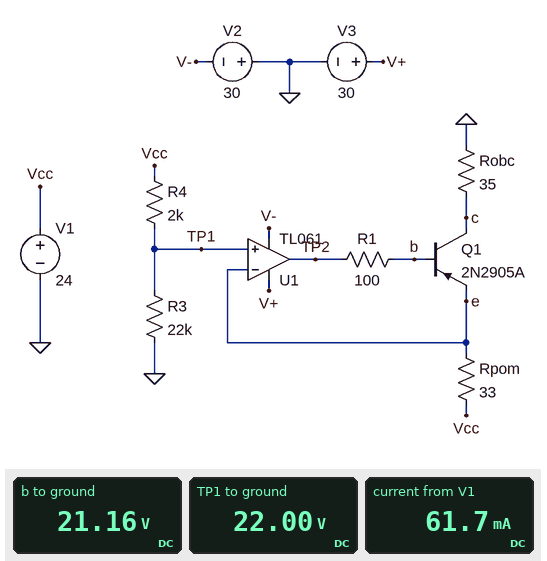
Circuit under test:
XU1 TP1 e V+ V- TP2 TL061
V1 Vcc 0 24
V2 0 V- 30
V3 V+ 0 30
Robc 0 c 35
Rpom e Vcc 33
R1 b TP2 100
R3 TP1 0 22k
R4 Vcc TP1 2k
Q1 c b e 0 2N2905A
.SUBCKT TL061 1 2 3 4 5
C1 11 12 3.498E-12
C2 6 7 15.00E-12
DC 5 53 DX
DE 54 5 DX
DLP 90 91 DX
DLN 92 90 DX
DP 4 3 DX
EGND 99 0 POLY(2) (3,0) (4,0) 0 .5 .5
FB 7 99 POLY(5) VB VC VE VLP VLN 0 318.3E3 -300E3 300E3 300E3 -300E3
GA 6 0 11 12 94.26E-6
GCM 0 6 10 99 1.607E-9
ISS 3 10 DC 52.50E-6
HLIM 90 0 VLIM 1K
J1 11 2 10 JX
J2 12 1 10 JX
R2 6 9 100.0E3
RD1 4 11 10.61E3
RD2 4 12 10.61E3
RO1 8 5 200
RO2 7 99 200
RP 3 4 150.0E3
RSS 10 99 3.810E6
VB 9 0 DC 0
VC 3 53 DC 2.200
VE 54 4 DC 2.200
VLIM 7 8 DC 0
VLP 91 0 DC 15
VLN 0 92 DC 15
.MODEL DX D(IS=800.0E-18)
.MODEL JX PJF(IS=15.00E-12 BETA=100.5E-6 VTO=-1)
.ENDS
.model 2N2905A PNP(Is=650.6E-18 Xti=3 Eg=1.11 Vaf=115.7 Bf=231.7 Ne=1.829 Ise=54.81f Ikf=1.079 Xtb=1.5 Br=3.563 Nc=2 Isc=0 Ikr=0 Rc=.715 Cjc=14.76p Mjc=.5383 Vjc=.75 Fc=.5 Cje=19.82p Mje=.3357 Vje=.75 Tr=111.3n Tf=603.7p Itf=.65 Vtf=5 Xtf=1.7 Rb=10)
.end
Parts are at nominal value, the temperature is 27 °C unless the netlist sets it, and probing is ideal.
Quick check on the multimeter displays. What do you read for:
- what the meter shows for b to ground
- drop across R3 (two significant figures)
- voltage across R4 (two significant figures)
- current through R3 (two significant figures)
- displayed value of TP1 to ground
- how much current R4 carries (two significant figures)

21.16 V
22 V
2.0 V
1.0 mA
22.00 V
1.0 mA
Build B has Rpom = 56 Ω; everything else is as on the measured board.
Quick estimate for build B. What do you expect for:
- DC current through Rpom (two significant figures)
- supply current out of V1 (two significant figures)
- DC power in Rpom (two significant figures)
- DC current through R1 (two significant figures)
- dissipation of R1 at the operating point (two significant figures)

36 mA
37 mA
72 mW
140 µA
1.9 µW
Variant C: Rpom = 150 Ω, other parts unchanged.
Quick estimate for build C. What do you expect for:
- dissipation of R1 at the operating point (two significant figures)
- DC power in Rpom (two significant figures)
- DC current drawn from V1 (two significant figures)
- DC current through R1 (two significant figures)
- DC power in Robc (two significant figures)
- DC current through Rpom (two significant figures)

250 nW
27 mW
14 mA
50 µA
6.2 mW
13 mA
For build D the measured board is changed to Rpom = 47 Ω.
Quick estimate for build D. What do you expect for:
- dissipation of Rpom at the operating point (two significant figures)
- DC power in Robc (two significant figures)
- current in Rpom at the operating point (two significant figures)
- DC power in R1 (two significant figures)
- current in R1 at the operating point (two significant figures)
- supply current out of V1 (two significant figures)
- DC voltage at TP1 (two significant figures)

85 mW
63 mW
43 mA
2.7 µW
160 µA
44 mA
22 V
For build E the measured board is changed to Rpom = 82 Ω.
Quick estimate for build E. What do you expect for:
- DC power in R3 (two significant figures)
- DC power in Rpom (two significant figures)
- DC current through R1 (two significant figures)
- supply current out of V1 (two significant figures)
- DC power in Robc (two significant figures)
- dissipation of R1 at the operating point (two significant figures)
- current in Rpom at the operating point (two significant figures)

22 mW
49 mW
92 µA
25 mA
21 mW
850 nW
24 mA
